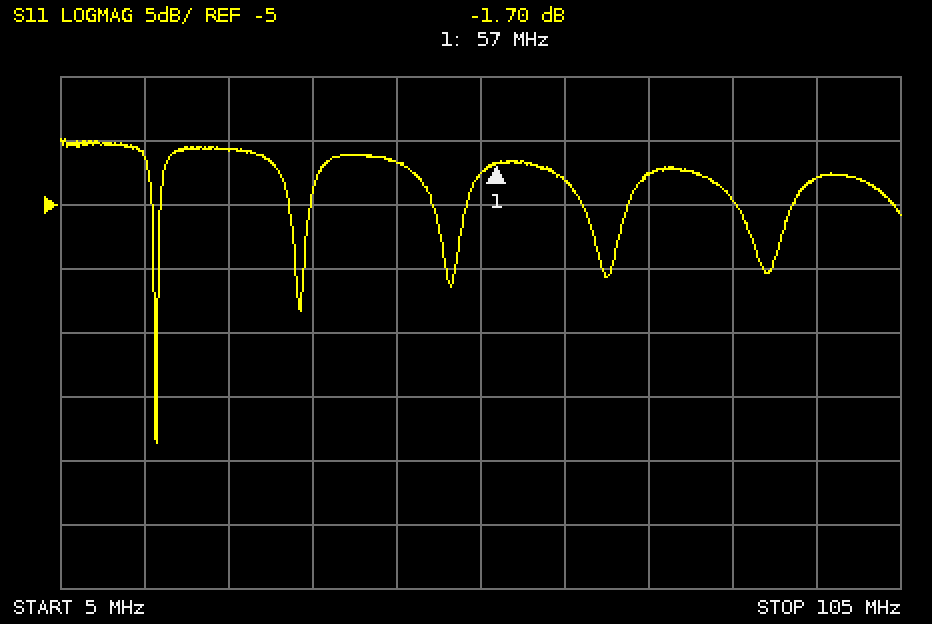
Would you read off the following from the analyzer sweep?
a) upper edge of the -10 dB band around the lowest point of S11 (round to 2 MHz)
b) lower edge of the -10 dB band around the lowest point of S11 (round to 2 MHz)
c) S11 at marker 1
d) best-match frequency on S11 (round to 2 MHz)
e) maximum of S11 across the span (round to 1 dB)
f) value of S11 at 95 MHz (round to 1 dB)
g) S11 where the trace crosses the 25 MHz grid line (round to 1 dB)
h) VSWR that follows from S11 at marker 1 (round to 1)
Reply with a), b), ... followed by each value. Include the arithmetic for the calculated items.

a) 16 MHz
b) 16 MHz
c) -1.70 dB
d) 16 MHz
e) 0 dB
f) -3 dB
g) -1 dB
h) (1 + 0.8222)/(1 − 0.8222) ≈ 10
